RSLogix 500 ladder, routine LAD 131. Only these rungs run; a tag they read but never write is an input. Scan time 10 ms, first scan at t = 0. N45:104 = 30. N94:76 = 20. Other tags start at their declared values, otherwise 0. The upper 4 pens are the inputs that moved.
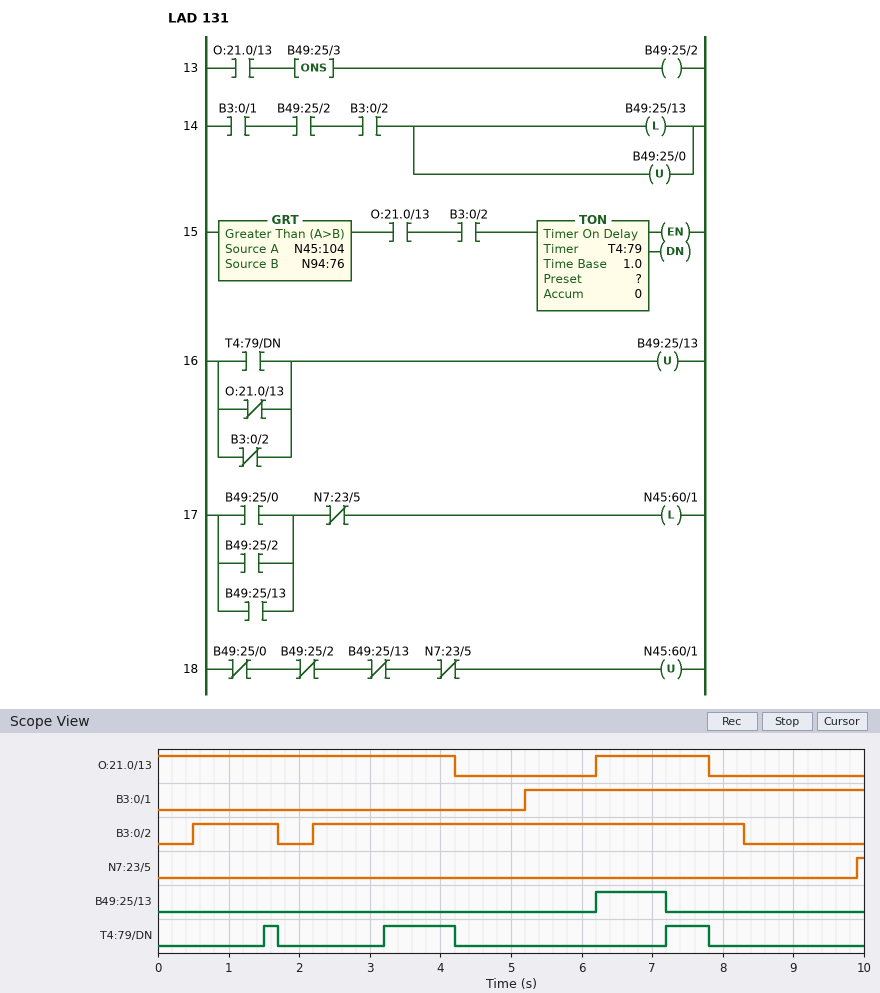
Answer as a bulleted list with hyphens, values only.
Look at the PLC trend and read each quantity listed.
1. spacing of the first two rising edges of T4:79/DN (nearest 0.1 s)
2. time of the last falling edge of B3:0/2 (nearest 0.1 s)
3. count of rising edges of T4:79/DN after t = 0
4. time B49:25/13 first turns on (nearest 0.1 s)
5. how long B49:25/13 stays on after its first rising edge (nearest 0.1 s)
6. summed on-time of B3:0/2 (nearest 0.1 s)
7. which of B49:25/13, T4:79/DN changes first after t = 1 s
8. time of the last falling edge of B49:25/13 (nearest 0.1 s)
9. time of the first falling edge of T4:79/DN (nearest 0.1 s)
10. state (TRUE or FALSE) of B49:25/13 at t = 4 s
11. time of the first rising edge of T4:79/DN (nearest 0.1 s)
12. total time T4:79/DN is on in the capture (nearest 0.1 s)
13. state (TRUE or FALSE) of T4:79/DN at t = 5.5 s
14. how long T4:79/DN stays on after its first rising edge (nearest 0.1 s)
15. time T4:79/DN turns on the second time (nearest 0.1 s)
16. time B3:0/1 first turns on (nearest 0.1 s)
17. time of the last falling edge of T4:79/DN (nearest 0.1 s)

- 1.7 s
- 8.3 s
- 3
- 6.2 s
- 1.0 s
- 7.3 s
- T4:79/DN
- 7.2 s
- 1.7 s
- FALSE
- 1.5 s
- 1.8 s
- FALSE
- 0.2 s
- 3.2 s
- 5.2 s
- 7.8 s
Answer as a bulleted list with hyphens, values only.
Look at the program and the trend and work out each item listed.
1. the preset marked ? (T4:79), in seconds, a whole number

- 1 s
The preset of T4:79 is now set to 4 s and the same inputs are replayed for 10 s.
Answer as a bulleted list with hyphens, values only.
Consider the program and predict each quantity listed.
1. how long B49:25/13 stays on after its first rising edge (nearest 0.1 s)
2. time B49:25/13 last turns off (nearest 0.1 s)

- 1.6 s
- 7.8 s
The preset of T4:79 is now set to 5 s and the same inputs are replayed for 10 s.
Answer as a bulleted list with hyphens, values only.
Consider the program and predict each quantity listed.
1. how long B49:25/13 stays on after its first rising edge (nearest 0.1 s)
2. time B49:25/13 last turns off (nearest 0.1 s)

- 1.6 s
- 7.8 s
